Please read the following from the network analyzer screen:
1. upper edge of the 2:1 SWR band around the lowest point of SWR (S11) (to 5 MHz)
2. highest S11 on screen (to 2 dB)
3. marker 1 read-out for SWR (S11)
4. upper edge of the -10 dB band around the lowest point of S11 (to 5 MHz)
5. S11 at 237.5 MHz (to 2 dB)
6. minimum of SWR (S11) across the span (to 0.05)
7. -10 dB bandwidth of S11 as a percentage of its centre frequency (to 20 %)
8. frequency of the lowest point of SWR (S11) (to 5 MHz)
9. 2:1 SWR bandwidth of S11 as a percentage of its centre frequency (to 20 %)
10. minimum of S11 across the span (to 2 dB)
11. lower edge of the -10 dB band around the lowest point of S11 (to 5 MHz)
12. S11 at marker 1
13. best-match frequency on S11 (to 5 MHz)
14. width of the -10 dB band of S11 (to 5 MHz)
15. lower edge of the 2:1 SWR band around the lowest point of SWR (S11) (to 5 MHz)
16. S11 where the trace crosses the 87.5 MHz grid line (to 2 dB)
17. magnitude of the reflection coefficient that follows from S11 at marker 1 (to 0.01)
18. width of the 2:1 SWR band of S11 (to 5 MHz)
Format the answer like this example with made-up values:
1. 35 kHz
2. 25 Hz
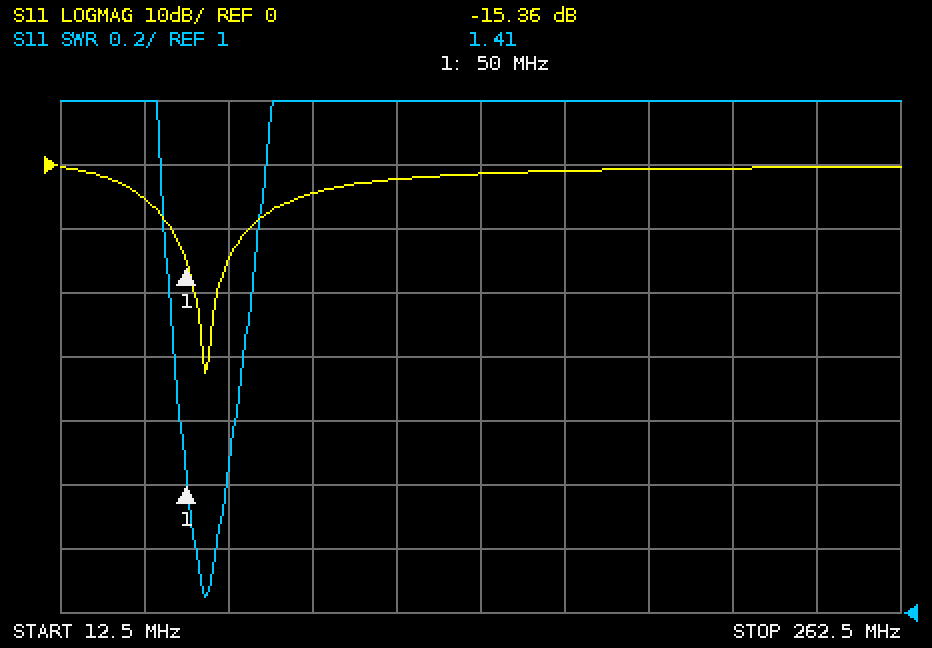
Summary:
1. 70 MHz
2. 0 dB
3. 1.41
4. 70 MHz
5. 0 dB
6. 1.05
7. 40 %
8. 55 MHz
9. 40 %
10. -32 dB
11. 45 MHz
12. -15.36 dB
13. 55 MHz
14. 25 MHz
15. 45 MHz
16. -4 dB
17. 0.17
18. 25 MHz
